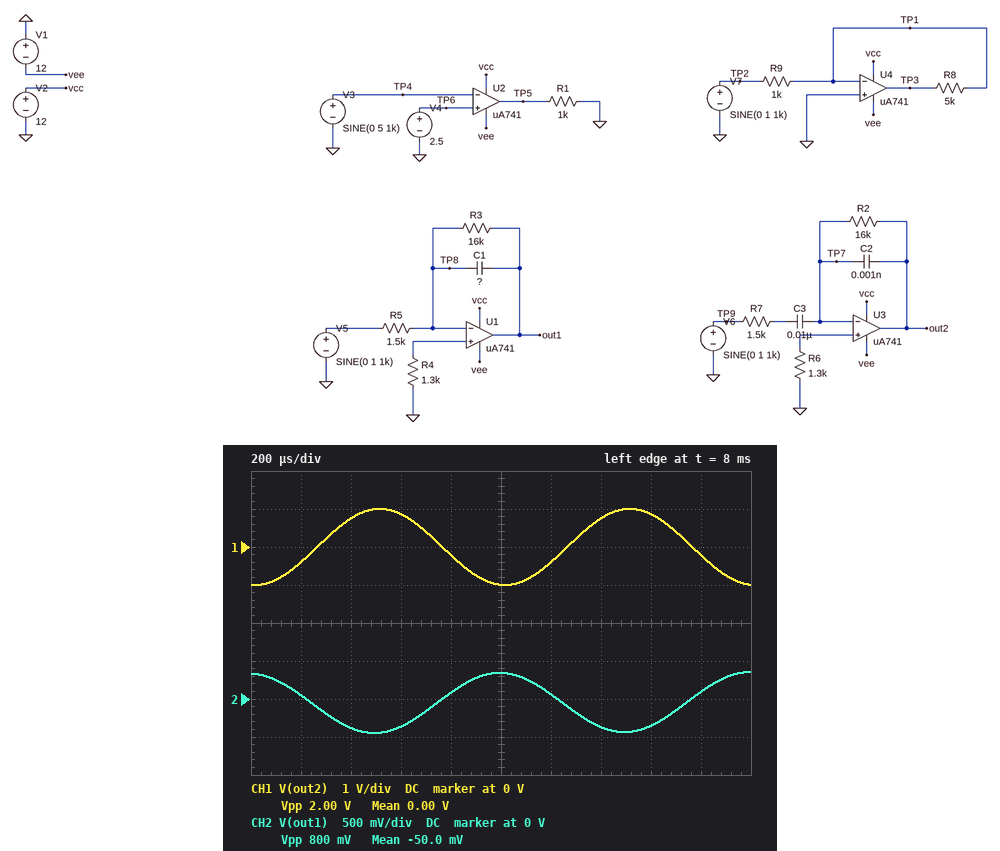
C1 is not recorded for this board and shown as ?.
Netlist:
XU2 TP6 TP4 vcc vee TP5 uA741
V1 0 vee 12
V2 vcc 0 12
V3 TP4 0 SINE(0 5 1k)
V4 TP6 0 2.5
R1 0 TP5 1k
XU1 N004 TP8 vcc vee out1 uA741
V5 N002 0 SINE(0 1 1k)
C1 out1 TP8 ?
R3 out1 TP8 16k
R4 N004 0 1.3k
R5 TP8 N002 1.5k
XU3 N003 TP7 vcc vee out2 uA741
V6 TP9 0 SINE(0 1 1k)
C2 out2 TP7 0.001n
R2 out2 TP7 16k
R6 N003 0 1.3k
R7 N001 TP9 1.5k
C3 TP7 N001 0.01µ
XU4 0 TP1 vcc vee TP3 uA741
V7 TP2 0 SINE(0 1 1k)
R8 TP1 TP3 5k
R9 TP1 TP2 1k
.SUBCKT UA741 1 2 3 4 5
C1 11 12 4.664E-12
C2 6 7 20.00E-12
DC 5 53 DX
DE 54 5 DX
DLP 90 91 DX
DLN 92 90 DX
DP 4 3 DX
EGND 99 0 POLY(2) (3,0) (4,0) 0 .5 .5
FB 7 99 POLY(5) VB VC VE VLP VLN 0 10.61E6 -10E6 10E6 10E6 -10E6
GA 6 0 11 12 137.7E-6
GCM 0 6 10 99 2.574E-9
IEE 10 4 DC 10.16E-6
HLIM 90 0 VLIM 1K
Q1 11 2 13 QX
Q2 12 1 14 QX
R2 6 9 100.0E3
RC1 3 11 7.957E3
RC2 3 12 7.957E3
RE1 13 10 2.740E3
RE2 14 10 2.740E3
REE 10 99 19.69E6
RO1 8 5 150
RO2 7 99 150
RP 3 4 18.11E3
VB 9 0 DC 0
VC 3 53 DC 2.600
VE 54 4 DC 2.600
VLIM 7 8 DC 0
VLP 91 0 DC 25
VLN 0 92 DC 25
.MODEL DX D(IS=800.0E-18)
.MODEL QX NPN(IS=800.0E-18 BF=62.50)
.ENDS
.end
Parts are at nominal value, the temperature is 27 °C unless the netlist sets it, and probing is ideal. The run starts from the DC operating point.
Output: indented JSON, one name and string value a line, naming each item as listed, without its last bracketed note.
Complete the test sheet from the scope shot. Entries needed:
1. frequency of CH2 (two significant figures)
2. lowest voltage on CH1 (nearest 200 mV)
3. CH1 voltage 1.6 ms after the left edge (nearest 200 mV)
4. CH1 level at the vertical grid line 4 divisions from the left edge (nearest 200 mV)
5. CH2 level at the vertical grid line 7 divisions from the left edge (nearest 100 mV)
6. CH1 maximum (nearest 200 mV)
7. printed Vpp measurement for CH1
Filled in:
{
  "frequency of CH2": "1.0 kHz",
  "lowest voltage on CH1": "-1.0 V",
  "CH1 voltage 1.6 ms after the left edge": "800 mV",
  "CH1 level at the vertical grid line 4 divisions from the left edge": "-200 mV",
  "CH2 level at the vertical grid line 7 divisions from the left edge": "-400 mV",
  "CH1 maximum": "1.0 V",
  "printed Vpp measurement for CH1": "2.00 V"
}
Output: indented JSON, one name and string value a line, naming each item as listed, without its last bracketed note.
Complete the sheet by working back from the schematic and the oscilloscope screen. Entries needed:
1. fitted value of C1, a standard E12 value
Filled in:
{
  "fitted value of C1, a standard E12 value": "270 nF"
}
